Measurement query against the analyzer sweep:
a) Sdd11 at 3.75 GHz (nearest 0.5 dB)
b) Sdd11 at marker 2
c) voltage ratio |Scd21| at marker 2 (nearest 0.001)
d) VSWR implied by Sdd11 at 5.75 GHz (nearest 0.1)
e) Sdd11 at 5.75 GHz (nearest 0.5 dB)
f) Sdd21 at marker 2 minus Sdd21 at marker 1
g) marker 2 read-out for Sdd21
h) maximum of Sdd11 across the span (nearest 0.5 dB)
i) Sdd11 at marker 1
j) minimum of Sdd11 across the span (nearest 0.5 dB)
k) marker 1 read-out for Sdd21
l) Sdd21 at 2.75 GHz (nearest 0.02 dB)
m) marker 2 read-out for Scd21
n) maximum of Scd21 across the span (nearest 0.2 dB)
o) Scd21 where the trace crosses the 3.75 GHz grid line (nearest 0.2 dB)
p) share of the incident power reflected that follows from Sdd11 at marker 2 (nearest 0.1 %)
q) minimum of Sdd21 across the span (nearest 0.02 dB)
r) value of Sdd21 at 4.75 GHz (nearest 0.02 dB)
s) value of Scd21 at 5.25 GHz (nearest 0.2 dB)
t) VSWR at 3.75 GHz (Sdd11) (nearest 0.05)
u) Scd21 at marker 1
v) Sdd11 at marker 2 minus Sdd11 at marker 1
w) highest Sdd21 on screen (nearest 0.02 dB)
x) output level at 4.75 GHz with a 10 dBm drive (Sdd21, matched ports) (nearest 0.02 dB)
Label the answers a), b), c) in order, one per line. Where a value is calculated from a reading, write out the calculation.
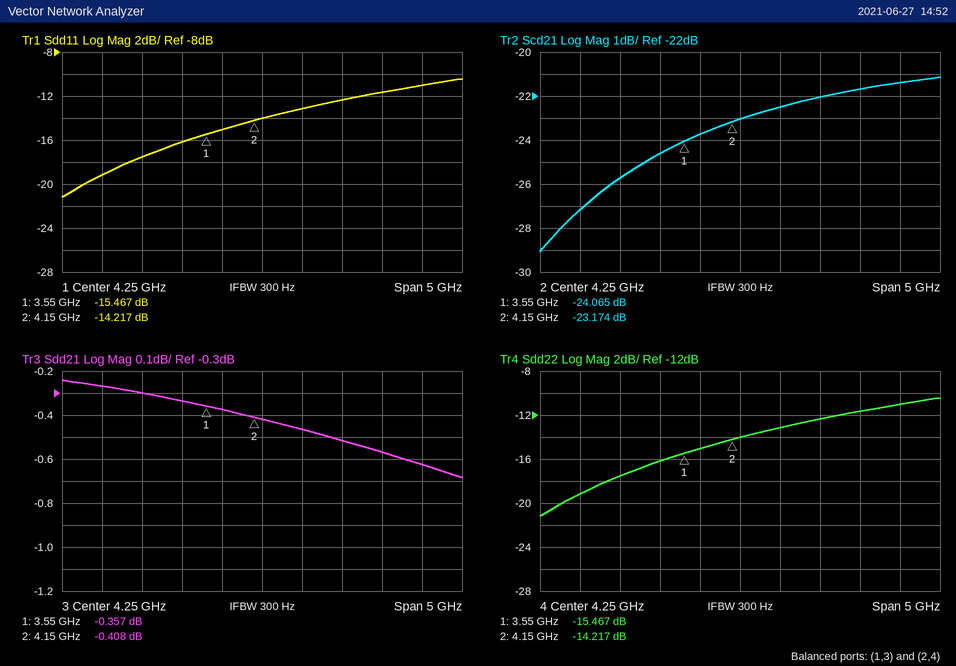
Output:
a) -15.0 dB
b) -14.217 dB
c) 10^(-23.174/20) ≈ 0.069
d) |Γ| = 10^(-11.5/20) = 0.2661; VSWR = (1 + 0.2661)/(1 − 0.2661) ≈ 1.7
e) -11.5 dB
f) -0.408 − (-0.357) = -0.051 dB
g) -0.408 dB
h) -10.5 dB
i) -15.467 dB
j) -21.0 dB
k) -0.357 dB
l) -0.30 dB
m) -23.174 dB
n) -21.2 dB
o) -23.8 dB
p) 10^(-14.217/10) ≈ 3.8 %
q) -0.68 dB
r) -0.46 dB
s) -22.0 dB
t) |Γ| = 10^(-15/20) = 0.1778; VSWR = (1 + 0.1778)/(1 − 0.1778) ≈ 1.43, so 1.45 to the nearest 0.05
u) -24.065 dB
v) -14.217 − (-15.467) = 1.250 dB
w) -0.24 dB
x) 10 dBm + (-0.46 dB) = 9.54 dBm
